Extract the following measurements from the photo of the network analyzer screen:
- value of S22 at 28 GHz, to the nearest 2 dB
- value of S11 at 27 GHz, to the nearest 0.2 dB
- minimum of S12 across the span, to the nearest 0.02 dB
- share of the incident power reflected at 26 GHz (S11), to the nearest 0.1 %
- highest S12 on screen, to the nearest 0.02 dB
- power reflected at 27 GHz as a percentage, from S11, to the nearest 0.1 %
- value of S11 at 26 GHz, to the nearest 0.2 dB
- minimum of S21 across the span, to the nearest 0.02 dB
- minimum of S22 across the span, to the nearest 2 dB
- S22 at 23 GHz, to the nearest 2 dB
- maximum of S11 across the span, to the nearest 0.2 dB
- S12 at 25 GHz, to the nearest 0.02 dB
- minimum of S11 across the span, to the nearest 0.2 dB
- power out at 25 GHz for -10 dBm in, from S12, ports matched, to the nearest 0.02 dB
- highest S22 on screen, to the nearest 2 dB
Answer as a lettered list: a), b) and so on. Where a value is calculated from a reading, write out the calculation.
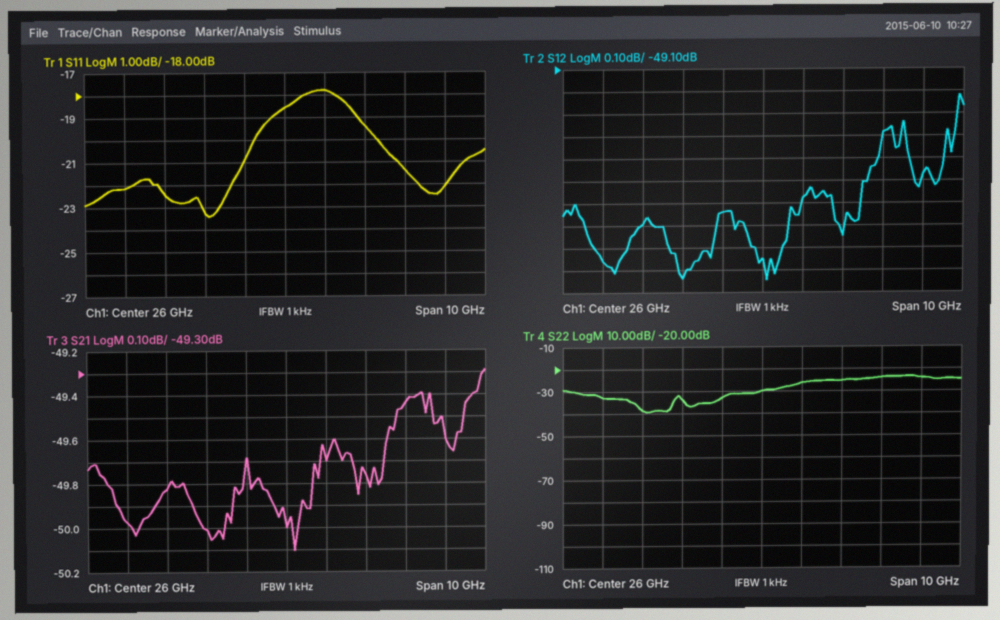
a) -26 dB
b) -17.8 dB
c) -50.04 dB
d) 10^(-18.6/10) ≈ 1.4 %
e) -49.22 dB
f) 10^(-17.8/10) ≈ 1.7 %
g) -18.6 dB
h) -50.10 dB
i) -40 dB
j) -38 dB
k) -17.8 dB
l) -49.74 dB
m) -23.4 dB
n) -10 dBm + (-49.74 dB) = -59.74 dBm
o) -24 dB
